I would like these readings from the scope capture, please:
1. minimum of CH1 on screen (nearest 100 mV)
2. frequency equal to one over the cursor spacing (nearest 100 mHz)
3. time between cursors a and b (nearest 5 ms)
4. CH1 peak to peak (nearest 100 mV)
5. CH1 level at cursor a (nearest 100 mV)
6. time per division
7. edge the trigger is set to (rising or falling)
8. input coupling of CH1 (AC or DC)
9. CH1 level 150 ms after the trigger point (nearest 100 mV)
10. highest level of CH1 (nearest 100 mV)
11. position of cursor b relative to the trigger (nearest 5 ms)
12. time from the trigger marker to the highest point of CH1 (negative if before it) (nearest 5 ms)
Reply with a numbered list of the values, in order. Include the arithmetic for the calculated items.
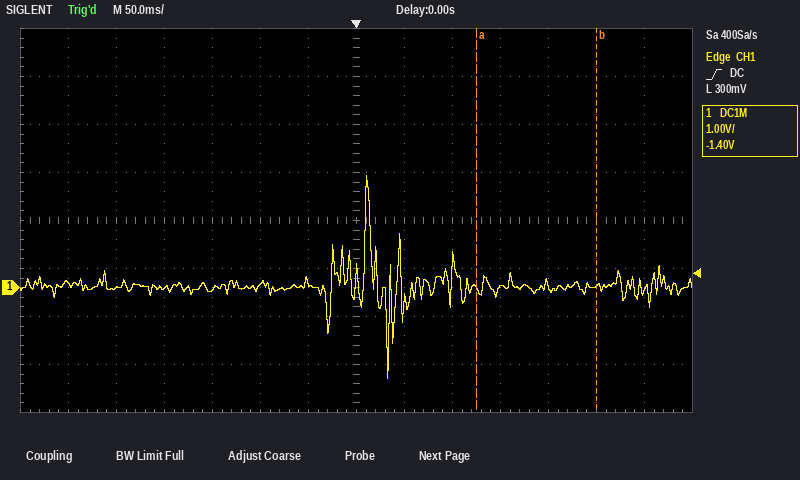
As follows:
1. -1.9 V
2. 1 / 125 ms ≈ 8.0 Hz
3. 125 ms
4. 2.3 V − (-1.9 V) = 4.2 V
5. 0.0 V
6. 50 ms
7. rising
8. DC
9. 0.0 V
10. 2.3 V
11. +250 ms
12. +10 ms
